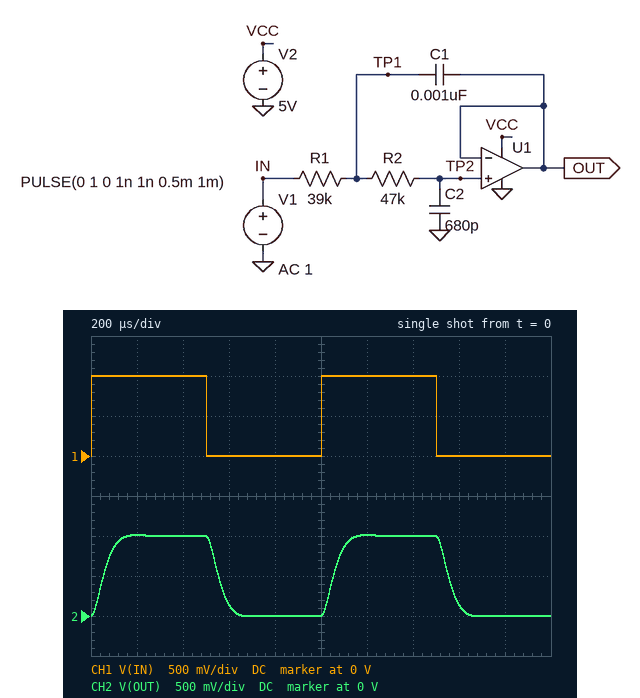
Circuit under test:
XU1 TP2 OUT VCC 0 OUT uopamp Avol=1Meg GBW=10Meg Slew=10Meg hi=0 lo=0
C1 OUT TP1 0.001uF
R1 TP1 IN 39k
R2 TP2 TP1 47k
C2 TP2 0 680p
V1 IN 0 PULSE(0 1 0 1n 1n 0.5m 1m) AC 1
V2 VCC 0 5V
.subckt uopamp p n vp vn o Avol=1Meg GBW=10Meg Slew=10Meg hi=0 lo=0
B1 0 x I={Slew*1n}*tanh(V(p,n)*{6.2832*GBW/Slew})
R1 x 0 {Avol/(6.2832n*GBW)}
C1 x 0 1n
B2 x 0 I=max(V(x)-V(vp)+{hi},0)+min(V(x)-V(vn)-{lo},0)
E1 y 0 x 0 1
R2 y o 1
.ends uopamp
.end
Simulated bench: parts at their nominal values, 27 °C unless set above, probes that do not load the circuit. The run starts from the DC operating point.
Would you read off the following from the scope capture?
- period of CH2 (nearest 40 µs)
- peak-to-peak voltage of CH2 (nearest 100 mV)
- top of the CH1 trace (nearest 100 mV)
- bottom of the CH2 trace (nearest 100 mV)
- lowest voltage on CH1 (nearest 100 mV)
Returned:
1.00 ms
1.0 V
1.0 V
0 V
0 V
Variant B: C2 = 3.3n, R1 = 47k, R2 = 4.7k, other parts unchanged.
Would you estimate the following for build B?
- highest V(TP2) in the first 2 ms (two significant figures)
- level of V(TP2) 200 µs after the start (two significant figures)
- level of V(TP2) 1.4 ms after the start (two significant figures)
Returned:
950 mV
690 mV
910 mV
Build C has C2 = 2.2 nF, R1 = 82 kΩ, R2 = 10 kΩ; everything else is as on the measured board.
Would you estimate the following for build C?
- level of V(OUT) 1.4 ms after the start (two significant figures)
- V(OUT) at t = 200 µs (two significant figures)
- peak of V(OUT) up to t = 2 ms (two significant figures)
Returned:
880 mV
630 mV
930 mV
